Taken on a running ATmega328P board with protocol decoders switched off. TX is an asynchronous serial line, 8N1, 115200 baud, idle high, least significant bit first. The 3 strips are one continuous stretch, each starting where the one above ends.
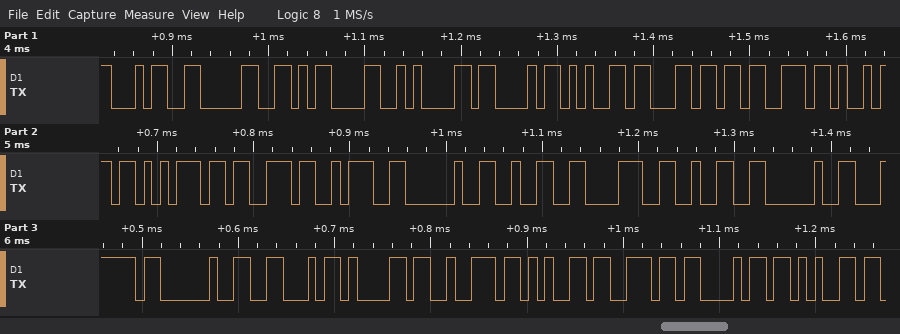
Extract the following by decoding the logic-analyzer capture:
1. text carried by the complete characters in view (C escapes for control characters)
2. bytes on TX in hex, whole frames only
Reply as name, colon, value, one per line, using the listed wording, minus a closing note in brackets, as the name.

text carried by the complete characters in view: "40\r\nCelsius: 282 | Farenhe"
bytes on TX in hex, whole frames only: 34 30 0D 0A 43 65 6C 73 69 75 73 3A 20 32 38 32 20 7C 20 46 61 72 65 6E 68 65
